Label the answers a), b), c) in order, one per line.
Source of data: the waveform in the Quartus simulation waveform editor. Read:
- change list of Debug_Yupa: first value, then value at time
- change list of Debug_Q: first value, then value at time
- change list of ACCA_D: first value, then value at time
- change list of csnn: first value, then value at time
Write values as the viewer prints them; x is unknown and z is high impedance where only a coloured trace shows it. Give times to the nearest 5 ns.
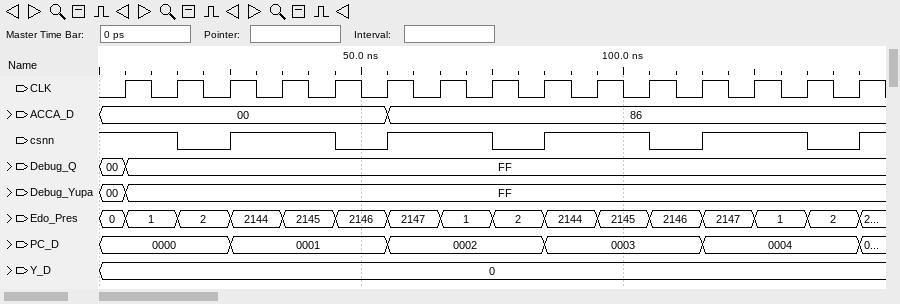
a) 00, FF at 5 ns
b) 00, FF at 5 ns
c) 00, 86 at 55 ns
d) 1, 0 at 15 ns, 1 at 25 ns, 0 at 45 ns, 1 at 55 ns, 0 at 75 ns, 1 at 85 ns, 0 at 105 ns, 1 at 115 ns, 0 at 135 ns, 1 at 145 ns
